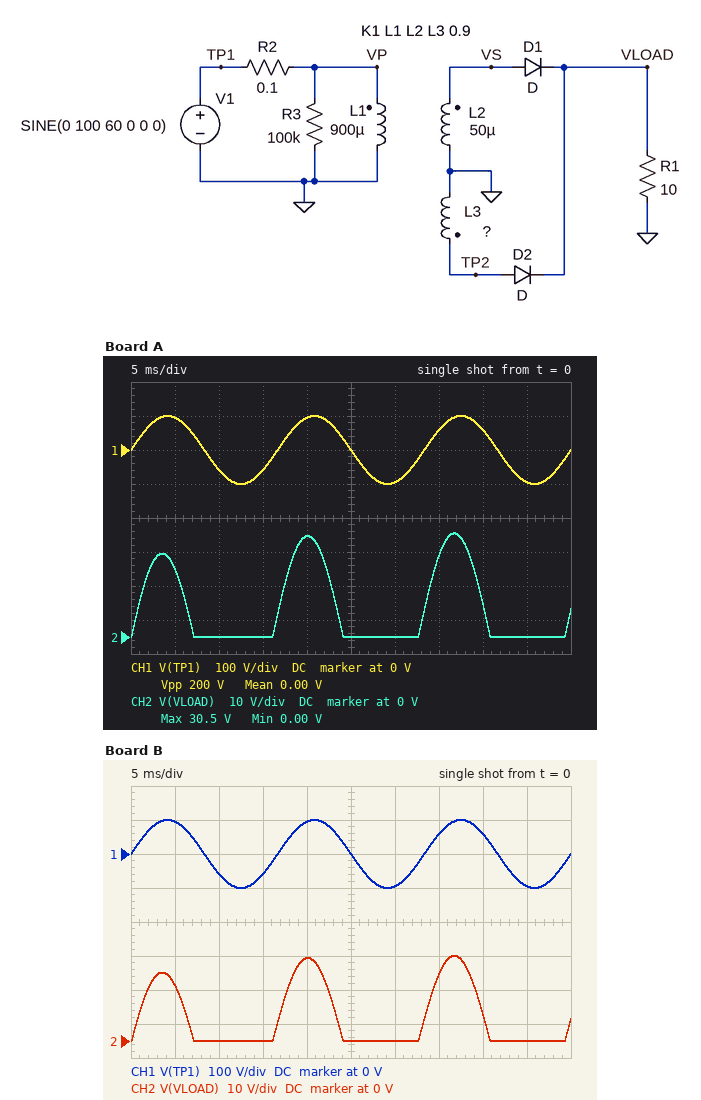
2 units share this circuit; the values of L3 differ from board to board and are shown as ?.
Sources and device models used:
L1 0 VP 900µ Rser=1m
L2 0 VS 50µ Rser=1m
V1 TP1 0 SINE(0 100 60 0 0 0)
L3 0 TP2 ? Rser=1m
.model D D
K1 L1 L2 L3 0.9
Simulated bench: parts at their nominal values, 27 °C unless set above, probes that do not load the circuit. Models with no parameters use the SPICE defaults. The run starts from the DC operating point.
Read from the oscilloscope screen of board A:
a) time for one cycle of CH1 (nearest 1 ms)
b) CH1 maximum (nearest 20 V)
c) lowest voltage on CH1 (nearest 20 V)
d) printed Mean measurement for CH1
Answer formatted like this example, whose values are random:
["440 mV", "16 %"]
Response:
["17 ms", "100 V", "-100 V", "0.00 V"]
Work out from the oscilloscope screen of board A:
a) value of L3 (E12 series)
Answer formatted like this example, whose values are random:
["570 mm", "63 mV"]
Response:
["120 µH"]
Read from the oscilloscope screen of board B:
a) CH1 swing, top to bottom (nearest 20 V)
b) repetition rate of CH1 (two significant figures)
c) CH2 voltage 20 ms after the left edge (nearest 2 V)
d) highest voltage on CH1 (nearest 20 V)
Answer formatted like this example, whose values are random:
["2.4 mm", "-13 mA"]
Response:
["200 V", "60 Hz", "24 V", "100 V"]
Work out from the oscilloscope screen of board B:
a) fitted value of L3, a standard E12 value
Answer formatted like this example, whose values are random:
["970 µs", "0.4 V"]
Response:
["82 µH"]
